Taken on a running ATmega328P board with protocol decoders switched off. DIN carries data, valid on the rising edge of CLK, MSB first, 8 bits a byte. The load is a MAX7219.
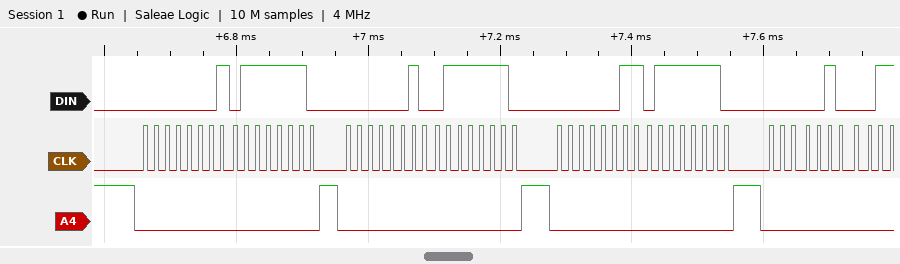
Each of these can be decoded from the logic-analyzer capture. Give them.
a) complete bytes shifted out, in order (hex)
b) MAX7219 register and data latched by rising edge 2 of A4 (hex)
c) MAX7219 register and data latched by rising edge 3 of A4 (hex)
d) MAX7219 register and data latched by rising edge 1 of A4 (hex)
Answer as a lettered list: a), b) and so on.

a) 01 7E 02 7E 03 7E 04
b) register 0x2, data 0x7E
c) register 0x3, data 0x7E
d) register 0x1, data 0x7E
